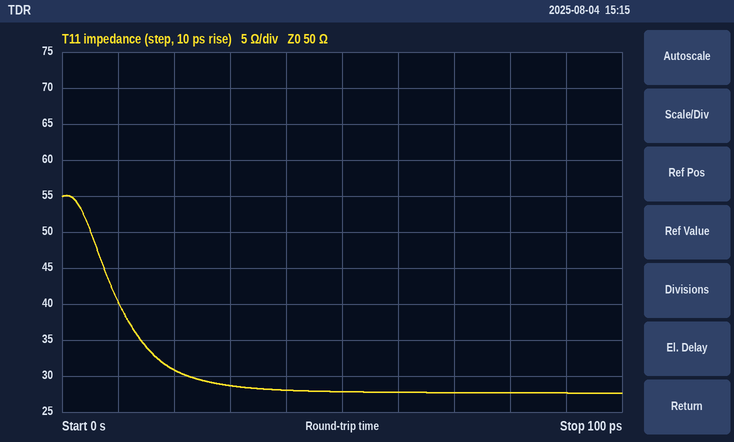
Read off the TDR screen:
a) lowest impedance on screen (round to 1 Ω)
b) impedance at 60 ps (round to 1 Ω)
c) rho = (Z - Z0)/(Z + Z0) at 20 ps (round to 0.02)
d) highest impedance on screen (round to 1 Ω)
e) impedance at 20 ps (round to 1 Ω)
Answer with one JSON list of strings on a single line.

["28 Ω", "28 Ω", "-0.24", "55 Ω", "31 Ω"]
